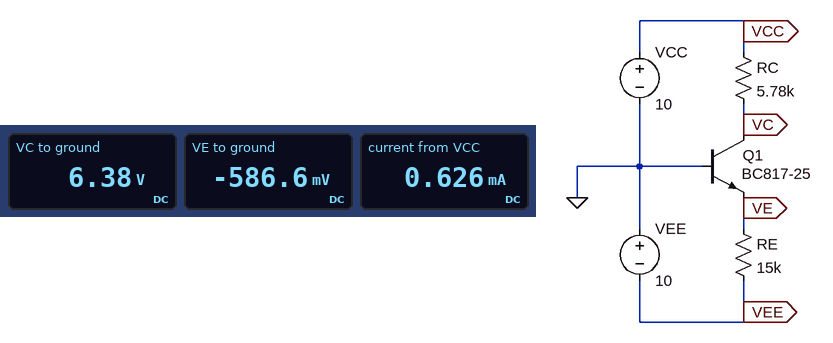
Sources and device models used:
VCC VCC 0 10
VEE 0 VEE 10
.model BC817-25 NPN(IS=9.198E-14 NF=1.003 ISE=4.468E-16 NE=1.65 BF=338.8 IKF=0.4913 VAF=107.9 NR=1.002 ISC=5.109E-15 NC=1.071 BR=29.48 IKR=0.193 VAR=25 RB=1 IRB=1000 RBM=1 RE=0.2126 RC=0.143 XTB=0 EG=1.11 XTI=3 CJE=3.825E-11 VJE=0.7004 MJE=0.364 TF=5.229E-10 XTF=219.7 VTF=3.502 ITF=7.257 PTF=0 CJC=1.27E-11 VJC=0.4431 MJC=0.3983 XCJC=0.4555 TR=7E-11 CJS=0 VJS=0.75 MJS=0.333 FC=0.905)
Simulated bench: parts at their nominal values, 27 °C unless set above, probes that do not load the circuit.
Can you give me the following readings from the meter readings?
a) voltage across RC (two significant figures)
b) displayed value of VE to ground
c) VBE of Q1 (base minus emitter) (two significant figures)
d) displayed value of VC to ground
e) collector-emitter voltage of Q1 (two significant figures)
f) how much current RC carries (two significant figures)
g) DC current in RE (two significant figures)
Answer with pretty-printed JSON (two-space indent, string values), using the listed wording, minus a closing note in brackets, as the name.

{
  "voltage across RC": "3.6 V",
  "displayed value of VE to ground": "-586.6 mV",
  "VBE of Q1 (base minus emitter)": "590 mV",
  "displayed value of VC to ground": "6.38 V",
  "collector-emitter voltage of Q1": "7.0 V",
  "how much current RC carries": "630 µA",
  "DC current in RE": "630 µA"
}
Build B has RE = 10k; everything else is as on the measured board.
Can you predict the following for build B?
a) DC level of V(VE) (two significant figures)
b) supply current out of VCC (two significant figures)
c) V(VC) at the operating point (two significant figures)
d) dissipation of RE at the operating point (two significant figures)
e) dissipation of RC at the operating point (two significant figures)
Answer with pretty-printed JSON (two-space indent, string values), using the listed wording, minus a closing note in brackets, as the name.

{
  "DC level of V(VE)": "-600 mV",
  "supply current out of VCC": "940 µA",
  "V(VC) at the operating point": "4.6 V",
  "dissipation of RE at the operating point": "8.8 mW",
  "dissipation of RC at the operating point": "5.1 mW"
}
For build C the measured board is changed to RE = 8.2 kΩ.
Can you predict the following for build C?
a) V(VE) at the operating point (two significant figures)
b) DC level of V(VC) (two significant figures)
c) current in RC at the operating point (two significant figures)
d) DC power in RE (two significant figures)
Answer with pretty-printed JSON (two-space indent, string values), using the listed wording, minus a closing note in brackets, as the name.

{
  "V(VE) at the operating point": "-600 mV",
  "DC level of V(VC)": "3.4 V",
  "current in RC at the operating point": "1.1 mA",
  "DC power in RE": "11 mW"
}
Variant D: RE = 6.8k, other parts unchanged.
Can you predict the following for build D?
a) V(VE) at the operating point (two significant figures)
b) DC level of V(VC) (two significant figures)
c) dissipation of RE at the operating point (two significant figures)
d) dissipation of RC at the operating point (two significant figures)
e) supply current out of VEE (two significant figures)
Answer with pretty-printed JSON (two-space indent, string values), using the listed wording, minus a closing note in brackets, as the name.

{
  "V(VE) at the operating point": "-610 mV",
  "DC level of V(VC)": "2.0 V",
  "dissipation of RE at the operating point": "13 mW",
  "dissipation of RC at the operating point": "11 mW",
  "supply current out of VEE": "1.4 mA"
}
